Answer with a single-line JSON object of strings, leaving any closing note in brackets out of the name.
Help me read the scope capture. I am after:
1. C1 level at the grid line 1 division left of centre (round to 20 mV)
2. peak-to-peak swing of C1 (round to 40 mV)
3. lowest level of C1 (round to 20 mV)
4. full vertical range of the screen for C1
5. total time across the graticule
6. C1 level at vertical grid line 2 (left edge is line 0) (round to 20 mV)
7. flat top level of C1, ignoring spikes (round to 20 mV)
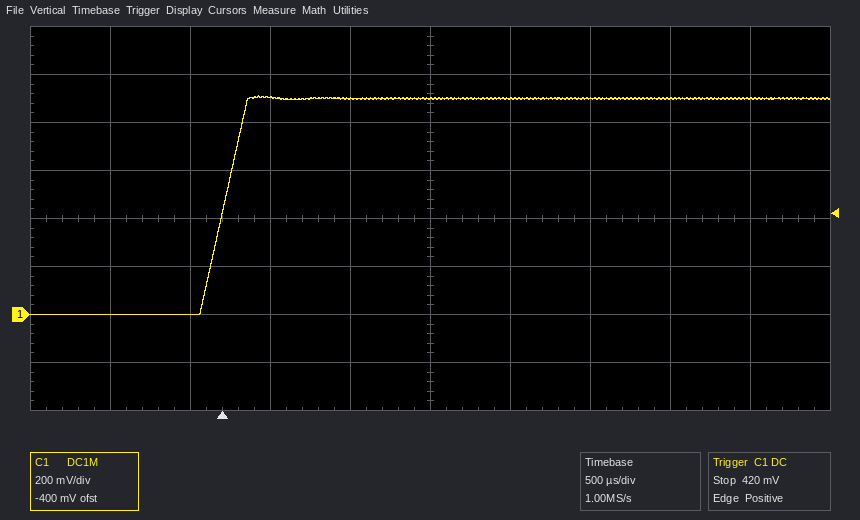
{"C1 level at the grid line 1 division left of centre": "900 mV", "peak-to-peak swing of C1": "920 mV", "lowest level of C1": "0 mV", "full vertical range of the screen for C1": "1.6 V", "total time across the graticule": "5 ms", "C1 level at vertical grid line 2 (left edge is line 0)": "0 mV", "flat top level of C1, ignoring spikes": "900 mV"}
